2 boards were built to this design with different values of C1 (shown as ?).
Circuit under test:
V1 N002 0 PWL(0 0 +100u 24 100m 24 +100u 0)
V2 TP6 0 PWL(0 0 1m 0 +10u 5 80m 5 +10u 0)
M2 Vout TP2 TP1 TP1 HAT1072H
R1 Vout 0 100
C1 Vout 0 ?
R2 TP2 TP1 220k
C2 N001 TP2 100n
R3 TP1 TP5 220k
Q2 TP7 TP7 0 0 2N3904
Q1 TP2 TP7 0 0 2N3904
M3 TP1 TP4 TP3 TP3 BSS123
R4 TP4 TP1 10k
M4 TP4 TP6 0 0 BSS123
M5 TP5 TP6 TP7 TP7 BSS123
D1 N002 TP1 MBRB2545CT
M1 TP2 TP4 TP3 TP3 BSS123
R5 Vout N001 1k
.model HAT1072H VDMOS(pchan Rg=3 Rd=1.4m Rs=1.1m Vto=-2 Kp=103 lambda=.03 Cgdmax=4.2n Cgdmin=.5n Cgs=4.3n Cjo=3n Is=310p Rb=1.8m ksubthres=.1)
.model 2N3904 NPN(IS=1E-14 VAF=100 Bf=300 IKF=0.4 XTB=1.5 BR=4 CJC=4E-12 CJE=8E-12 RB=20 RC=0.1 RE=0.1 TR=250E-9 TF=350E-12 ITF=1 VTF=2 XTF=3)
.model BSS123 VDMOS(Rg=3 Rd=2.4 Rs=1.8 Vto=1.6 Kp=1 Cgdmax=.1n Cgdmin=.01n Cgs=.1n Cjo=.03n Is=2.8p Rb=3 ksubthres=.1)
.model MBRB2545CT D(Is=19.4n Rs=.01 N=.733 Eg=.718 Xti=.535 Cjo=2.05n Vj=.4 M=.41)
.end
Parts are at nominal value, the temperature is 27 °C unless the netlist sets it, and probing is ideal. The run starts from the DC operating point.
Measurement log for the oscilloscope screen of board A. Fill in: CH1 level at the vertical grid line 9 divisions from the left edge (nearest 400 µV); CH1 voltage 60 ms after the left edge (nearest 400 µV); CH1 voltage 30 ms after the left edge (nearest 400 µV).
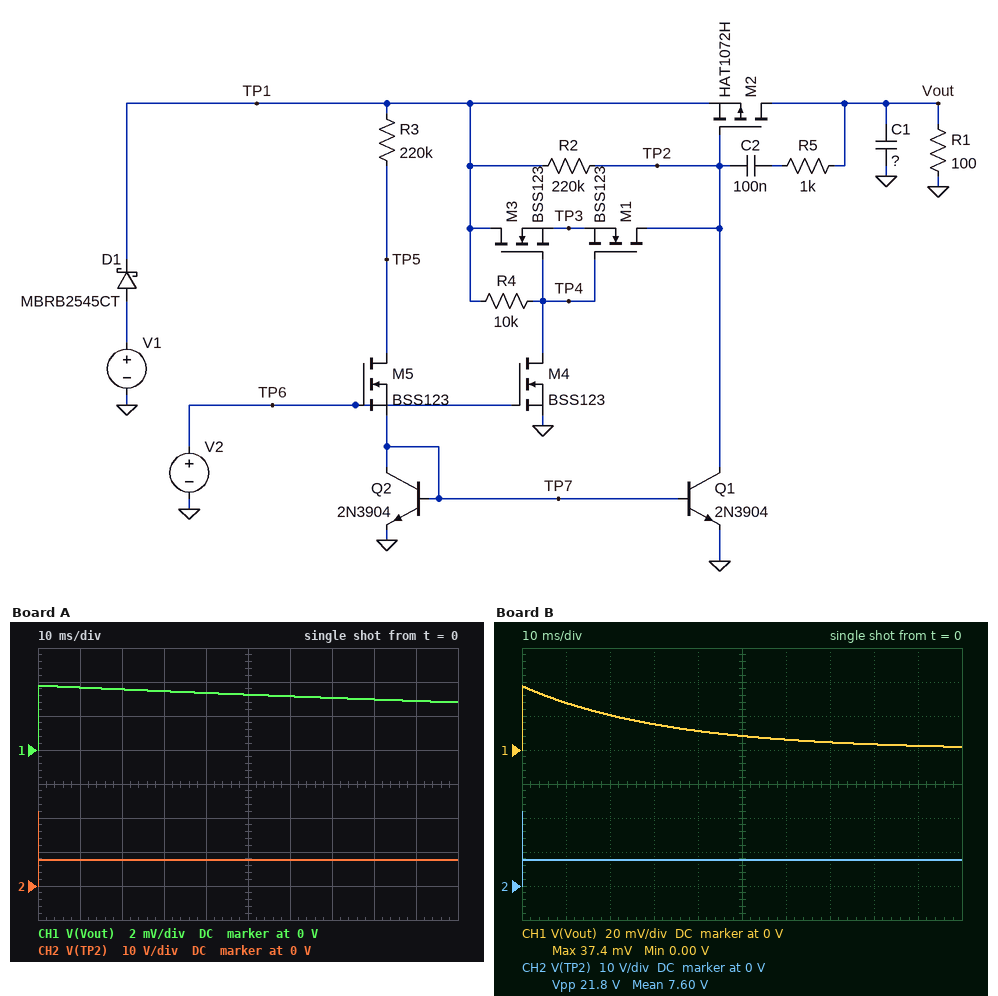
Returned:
2.8 mV
3.2 mV
3.6 mV
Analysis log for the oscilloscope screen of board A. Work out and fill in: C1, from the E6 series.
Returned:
3.3 mF
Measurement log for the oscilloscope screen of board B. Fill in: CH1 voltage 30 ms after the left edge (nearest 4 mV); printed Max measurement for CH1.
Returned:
16 mV
37.4 mV
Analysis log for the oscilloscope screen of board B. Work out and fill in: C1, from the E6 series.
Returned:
330 µF
